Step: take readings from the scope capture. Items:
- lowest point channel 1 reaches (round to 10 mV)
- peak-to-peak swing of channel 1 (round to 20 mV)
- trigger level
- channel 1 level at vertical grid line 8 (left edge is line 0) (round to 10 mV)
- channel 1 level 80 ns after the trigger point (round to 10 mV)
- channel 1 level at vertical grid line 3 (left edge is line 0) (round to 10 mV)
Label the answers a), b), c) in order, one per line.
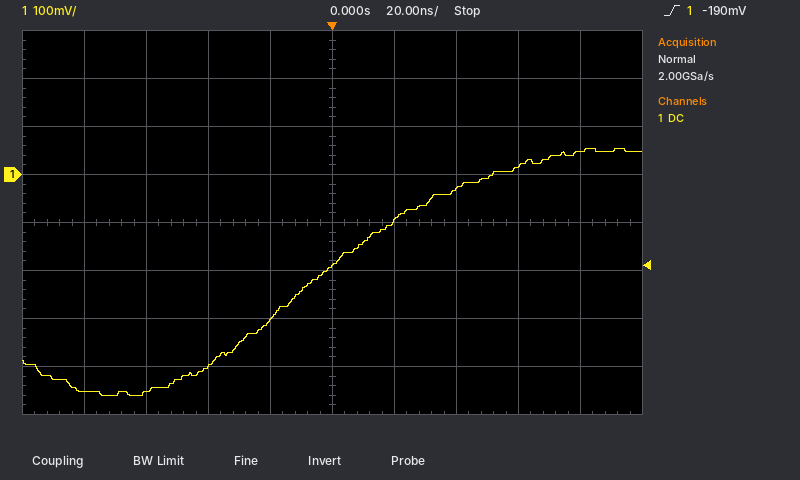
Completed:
a) -460 mV
b) 520 mV
c) -190 mV
d) 20 mV
e) 50 mV
f) -400 mV
